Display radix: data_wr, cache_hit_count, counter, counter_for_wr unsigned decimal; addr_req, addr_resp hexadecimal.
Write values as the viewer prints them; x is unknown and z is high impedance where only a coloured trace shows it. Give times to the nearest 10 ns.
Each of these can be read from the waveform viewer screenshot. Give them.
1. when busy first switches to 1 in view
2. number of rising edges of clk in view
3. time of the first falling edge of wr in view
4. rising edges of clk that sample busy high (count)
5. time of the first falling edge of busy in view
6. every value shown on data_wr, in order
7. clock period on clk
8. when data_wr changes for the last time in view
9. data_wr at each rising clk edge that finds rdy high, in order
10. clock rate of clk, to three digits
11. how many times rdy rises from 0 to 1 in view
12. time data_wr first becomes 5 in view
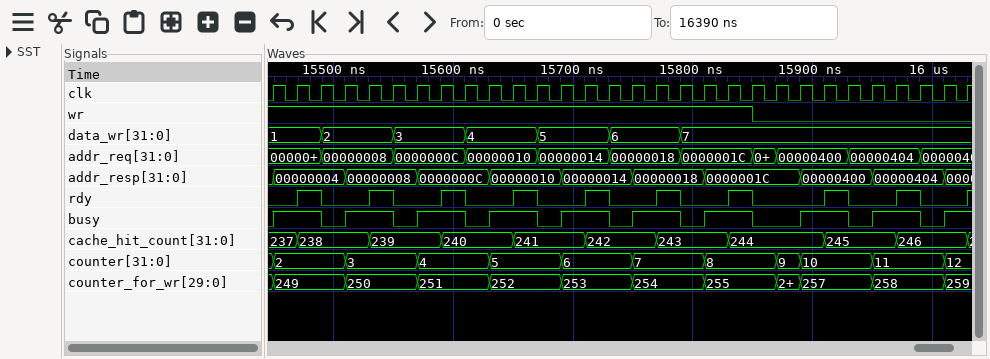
15450 ns
30
15850 ns
19
15490 ns
1, 2, 3, 4, 5, 6, 7
20 ns
15790 ns
1, 2, 3, 4, 5, 6, 7, 7, 7
50.0 MHz
10
15670 ns
